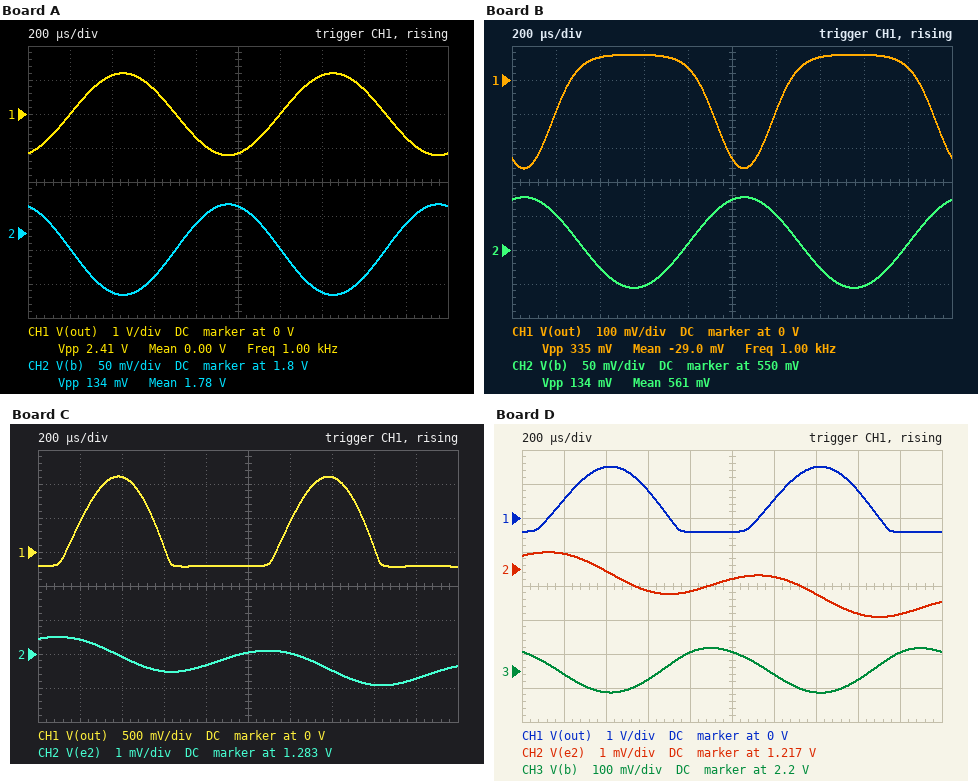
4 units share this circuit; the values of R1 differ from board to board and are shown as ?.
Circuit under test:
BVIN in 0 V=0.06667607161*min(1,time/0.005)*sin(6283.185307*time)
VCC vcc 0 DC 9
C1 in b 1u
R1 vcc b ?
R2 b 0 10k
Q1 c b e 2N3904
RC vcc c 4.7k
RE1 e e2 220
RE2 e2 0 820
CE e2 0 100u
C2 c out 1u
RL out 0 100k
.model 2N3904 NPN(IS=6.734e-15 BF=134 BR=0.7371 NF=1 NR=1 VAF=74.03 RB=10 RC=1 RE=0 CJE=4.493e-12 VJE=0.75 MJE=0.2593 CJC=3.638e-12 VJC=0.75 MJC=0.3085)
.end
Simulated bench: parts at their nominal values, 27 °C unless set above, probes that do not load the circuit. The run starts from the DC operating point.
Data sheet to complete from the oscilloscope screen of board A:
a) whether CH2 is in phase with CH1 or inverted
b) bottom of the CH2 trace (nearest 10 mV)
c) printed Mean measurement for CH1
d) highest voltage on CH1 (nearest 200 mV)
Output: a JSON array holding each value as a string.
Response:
["inverted", "1.71 V", "0.00 V", "1.2 V"]
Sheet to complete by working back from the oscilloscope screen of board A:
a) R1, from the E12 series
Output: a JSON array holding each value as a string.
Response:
["39 kΩ"]
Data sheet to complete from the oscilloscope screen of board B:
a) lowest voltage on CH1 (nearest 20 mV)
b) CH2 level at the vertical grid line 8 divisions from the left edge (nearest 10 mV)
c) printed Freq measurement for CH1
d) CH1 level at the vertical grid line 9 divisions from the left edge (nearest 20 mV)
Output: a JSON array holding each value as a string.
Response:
["-260 mV", "500 mV", "1.00 kHz", "40 mV"]
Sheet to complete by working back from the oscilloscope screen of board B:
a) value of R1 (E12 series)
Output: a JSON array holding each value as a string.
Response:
["150 kΩ"]
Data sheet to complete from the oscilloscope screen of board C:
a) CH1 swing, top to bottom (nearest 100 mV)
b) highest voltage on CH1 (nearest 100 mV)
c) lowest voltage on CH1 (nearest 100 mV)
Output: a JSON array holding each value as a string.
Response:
["1.3 V", "1.1 V", "-200 mV"]
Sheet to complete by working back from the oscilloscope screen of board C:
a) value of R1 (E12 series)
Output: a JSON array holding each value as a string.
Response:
["22 kΩ"]
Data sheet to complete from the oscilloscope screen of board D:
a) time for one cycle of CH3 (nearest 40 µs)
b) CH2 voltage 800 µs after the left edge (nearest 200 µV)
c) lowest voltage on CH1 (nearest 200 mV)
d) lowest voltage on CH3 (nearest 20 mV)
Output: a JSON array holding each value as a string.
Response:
["1.00 ms", "1.2164 V", "-400 mV", "2.14 V"]
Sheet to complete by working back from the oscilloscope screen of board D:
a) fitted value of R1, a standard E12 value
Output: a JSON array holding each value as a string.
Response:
["27 kΩ"]
